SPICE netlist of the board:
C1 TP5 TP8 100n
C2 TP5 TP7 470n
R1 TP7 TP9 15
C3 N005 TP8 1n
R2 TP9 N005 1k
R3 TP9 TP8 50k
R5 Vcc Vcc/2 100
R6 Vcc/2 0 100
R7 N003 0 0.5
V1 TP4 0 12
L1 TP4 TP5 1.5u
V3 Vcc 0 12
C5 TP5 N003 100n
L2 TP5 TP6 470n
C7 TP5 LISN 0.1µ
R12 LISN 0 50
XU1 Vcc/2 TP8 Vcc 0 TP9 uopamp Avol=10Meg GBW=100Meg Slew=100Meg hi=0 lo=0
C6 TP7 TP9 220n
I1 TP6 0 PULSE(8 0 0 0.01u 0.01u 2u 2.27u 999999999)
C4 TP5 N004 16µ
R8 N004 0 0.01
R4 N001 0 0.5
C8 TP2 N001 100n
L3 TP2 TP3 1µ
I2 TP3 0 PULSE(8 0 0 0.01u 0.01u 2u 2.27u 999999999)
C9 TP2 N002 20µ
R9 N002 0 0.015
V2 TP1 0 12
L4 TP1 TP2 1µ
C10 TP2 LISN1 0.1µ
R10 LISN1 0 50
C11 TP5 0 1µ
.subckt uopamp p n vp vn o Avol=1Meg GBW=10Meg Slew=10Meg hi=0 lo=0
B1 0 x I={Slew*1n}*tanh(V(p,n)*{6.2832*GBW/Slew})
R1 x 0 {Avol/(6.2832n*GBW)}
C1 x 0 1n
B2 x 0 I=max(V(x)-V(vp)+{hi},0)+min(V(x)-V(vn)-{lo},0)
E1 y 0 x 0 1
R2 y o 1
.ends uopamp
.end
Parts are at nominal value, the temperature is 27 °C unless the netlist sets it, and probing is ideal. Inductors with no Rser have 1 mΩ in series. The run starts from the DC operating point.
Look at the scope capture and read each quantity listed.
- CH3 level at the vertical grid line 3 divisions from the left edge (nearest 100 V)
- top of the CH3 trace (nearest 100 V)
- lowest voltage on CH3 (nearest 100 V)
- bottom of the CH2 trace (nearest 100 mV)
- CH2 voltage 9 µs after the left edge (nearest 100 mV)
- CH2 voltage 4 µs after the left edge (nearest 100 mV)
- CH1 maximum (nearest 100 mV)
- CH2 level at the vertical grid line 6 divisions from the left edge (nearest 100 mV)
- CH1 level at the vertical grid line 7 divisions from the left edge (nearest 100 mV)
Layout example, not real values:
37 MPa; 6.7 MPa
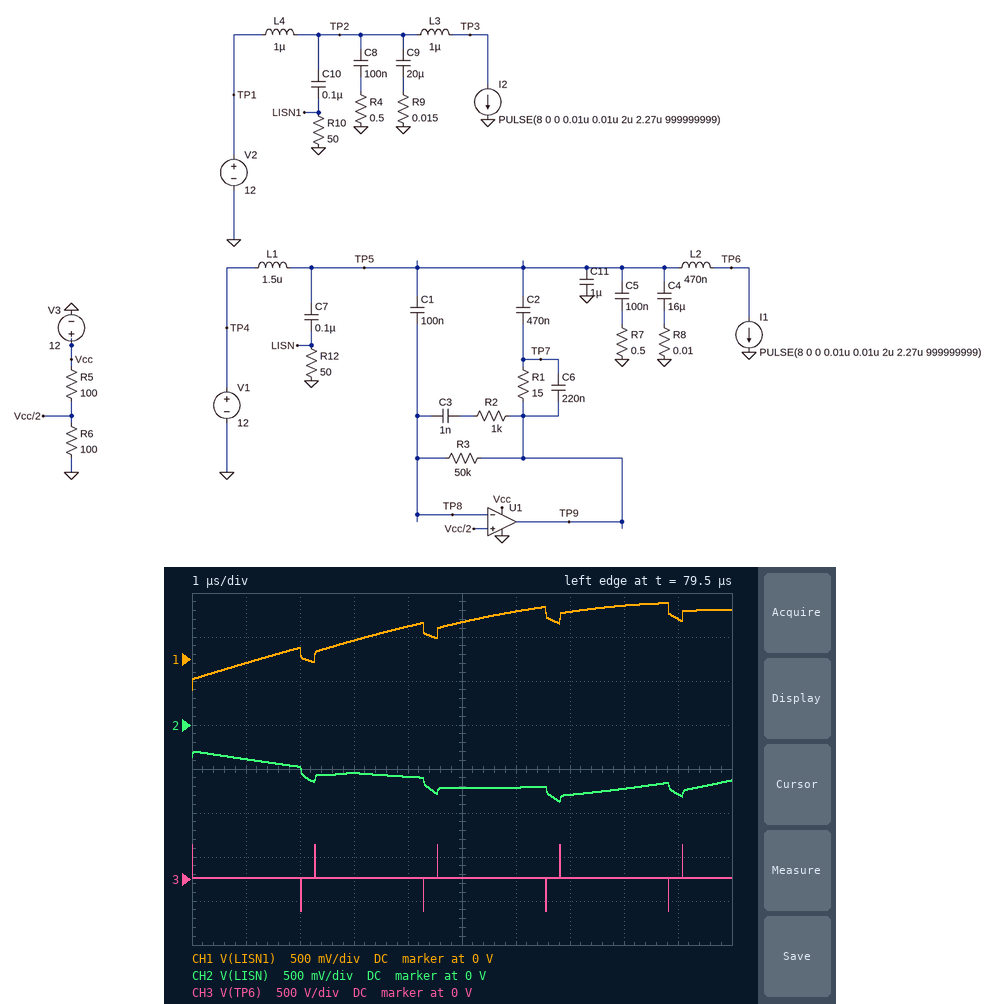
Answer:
0 V; 400 V; -400 V; -900 mV; -800 mV; -600 mV; 600 mV; -700 mV; 500 mV
